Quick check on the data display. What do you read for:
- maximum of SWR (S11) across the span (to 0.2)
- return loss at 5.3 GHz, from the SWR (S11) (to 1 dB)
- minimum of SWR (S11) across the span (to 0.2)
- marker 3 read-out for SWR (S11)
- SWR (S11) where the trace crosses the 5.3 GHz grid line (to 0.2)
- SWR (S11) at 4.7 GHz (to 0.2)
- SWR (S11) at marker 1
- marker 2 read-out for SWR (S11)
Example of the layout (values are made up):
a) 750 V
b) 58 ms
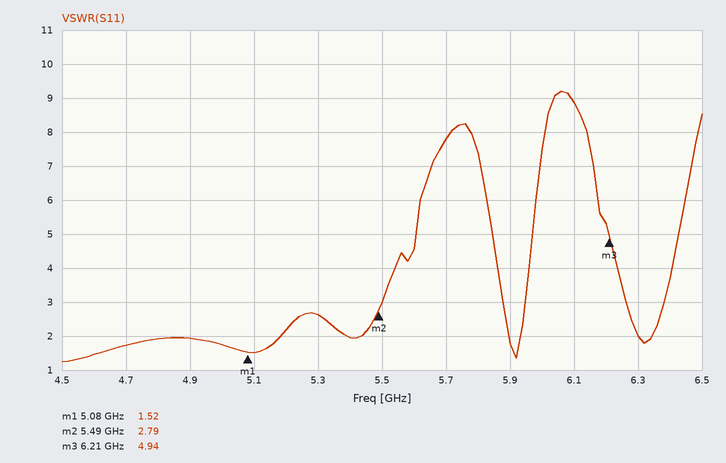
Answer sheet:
a) 9.2
b) 7 dB
c) 1.2
d) 4.94
e) 2.6
f) 1.8
g) 1.52
h) 2.79
